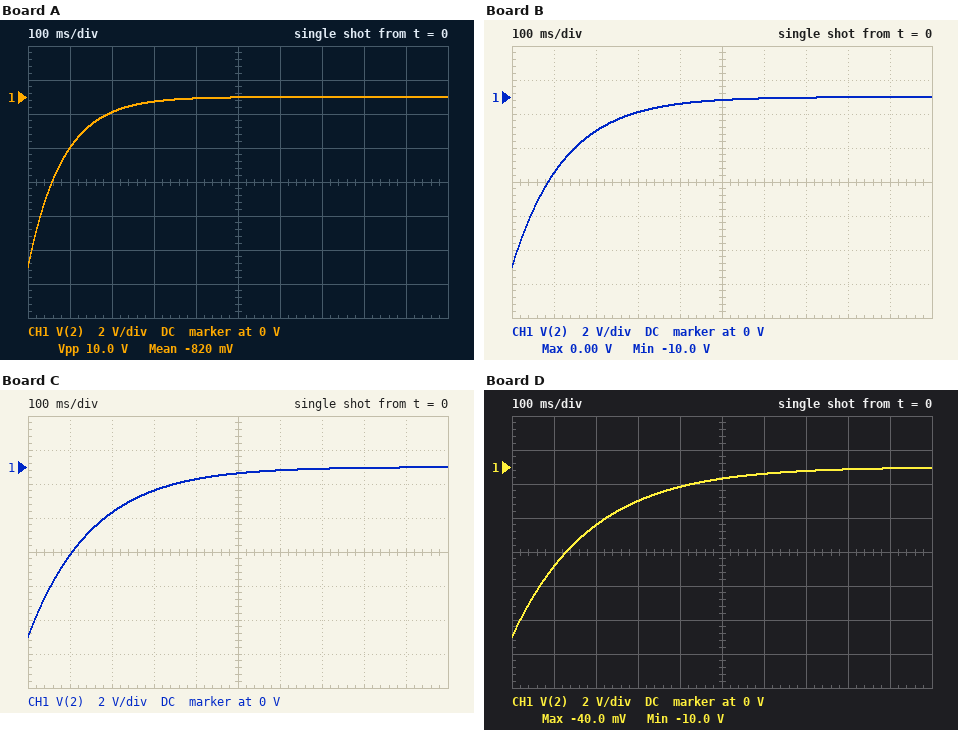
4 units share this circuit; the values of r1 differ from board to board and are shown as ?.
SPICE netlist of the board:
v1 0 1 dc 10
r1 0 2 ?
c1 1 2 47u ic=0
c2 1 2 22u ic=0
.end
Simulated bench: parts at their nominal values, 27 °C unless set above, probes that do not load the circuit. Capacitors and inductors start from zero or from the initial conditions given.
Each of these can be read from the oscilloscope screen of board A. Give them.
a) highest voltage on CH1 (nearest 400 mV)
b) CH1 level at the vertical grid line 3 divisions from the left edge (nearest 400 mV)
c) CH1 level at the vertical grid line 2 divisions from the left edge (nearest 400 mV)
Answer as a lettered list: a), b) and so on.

a) 0 V
b) -400 mV
c) -800 mV
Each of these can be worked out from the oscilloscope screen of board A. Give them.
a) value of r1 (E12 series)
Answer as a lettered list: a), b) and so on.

a) 1.2 kΩ
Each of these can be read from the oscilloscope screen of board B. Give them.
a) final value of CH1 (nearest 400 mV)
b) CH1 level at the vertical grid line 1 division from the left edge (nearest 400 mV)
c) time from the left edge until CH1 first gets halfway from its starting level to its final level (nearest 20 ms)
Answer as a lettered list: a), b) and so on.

a) 0 V
b) -4.4 V
c) 80 ms
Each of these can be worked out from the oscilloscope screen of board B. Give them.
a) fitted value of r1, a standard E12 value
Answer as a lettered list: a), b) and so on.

a) 1.8 kΩ
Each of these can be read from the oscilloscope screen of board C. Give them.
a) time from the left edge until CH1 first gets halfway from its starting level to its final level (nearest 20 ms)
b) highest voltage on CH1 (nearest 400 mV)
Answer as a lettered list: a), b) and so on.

a) 100 ms
b) 0 V
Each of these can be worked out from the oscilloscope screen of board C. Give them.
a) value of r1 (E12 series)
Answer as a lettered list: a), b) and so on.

a) 2.2 kΩ
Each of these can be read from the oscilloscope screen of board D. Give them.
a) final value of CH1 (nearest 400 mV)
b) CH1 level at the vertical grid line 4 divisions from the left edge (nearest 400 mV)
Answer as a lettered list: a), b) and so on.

a) 0 V
b) -1.2 V
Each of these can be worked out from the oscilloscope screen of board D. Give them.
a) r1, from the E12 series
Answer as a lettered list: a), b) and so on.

a) 2.7 kΩ
